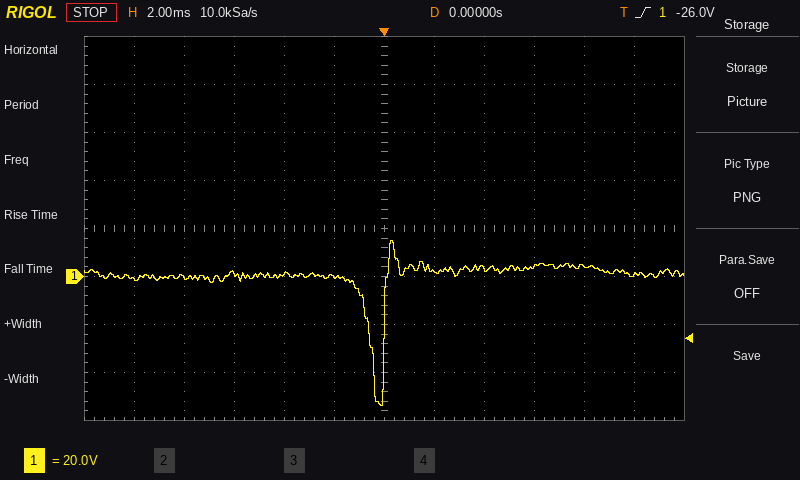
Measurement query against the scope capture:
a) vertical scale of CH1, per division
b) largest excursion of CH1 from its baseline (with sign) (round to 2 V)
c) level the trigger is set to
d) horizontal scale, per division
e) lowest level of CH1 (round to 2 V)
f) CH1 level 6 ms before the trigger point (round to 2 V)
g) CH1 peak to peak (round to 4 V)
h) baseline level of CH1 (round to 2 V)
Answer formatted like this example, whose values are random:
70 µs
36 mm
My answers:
20 V
-54 V
-26.0 V
2 ms
-54 V
2 V
68 V
0 V
